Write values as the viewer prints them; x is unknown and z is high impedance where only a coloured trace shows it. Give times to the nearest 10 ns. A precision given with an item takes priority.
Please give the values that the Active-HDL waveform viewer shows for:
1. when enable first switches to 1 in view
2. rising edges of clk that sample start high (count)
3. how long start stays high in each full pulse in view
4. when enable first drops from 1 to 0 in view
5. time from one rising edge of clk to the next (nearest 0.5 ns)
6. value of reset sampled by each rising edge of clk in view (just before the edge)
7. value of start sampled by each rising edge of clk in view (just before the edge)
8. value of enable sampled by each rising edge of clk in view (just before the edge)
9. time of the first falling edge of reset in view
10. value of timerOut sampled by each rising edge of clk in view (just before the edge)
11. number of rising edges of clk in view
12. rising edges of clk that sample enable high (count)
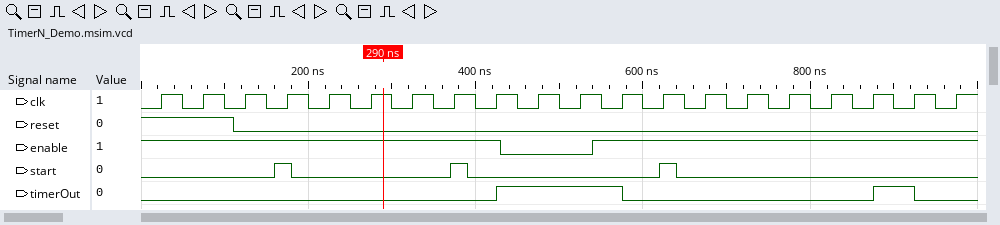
540 ns
3
20 ns, 20 ns, 20 ns
430 ns
50 ns
1 1 0 0 0 0 0 0 0 0 0 0 0 0 0 0 0 0 0 0
0 0 0 1 0 0 0 1 0 0 0 0 1 0 0 0 0 0 0 0
1 1 1 1 1 1 1 1 1 0 0 1 1 1 1 1 1 1 1 1
110 ns
0 0 0 0 0 0 0 0 0 1 1 1 0 0 0 0 0 0 1 0
20
18
